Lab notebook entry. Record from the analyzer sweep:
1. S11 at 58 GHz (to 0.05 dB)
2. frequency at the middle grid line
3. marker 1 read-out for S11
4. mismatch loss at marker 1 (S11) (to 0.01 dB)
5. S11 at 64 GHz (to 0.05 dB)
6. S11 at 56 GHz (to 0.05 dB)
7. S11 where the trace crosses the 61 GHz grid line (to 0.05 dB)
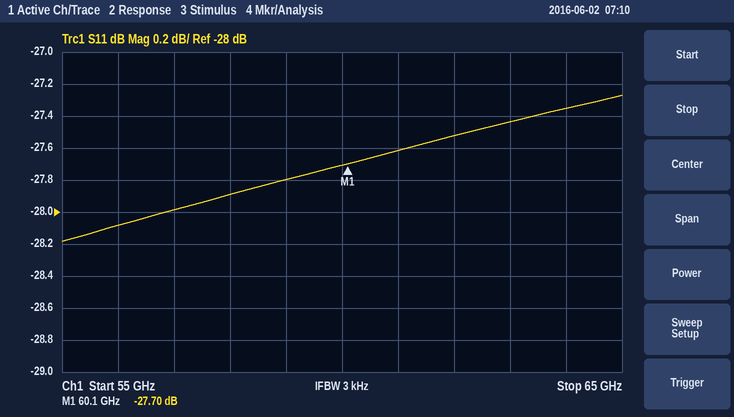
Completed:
-27.90 dB
60 GHz
-27.70 dB
0.01 dB
-27.35 dB
-28.10 dB
-27.60 dB
